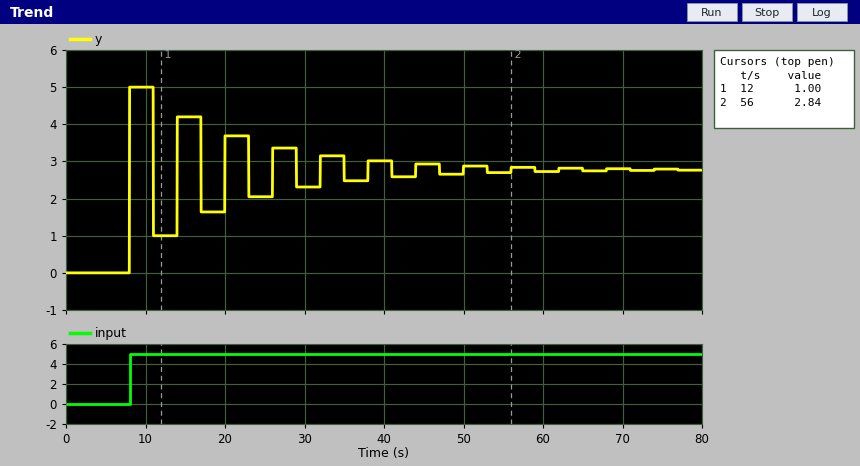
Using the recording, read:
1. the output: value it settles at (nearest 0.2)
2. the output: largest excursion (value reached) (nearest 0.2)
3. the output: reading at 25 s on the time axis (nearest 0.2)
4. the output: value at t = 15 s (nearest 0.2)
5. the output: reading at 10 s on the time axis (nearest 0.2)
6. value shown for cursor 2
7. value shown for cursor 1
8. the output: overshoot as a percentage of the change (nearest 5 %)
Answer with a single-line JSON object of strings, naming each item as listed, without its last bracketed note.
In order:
{"the output: value it settles at": "2.8", "the output: largest excursion (value reached)": "5.0", "the output: reading at 25 s on the time axis": "2.0", "the output: value at t = 15 s": "4.2", "the output: reading at 10 s on the time axis": "5.0", "value shown for cursor 2": "2.84", "value shown for cursor 1": "1.00", "the output: overshoot as a percentage of the change": "80 %"}
